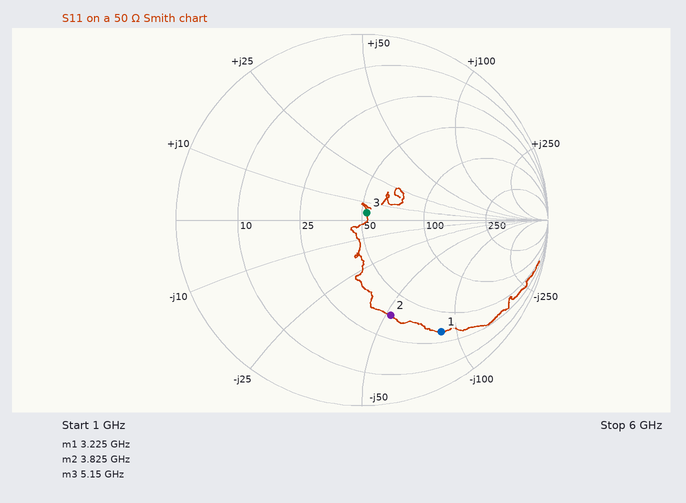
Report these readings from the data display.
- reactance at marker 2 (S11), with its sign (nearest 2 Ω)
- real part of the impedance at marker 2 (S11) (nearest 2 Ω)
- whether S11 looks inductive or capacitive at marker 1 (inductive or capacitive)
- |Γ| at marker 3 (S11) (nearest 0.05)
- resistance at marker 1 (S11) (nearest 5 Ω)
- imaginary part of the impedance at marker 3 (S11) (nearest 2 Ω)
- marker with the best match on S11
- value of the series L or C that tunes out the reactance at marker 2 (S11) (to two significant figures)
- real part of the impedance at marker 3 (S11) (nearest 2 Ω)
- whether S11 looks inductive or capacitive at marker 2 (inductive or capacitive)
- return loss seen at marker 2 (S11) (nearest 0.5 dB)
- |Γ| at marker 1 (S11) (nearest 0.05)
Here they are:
-52 Ω
36 Ω
capacitive
0.05
35 Ω
+4 Ω
marker 3
2.2 nH
52 Ω
capacitive
5.5 dB
0.75
